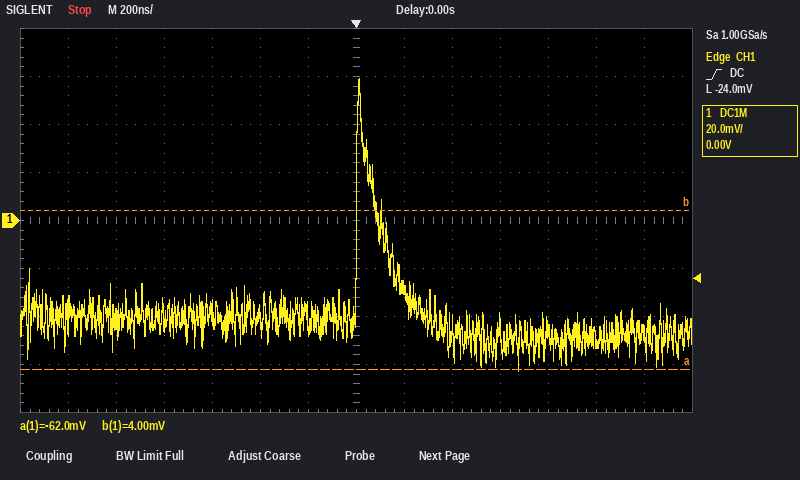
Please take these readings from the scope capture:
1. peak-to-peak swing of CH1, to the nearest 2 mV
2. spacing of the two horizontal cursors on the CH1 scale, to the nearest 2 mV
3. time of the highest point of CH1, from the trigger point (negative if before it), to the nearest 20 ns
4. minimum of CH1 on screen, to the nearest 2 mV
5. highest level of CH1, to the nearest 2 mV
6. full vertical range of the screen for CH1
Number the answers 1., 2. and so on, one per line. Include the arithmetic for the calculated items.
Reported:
1. 60 mV − (-62 mV) = 122 mV
2. 66 mV
3. +20 ns
4. -62 mV
5. 60 mV
6. 160 mV
